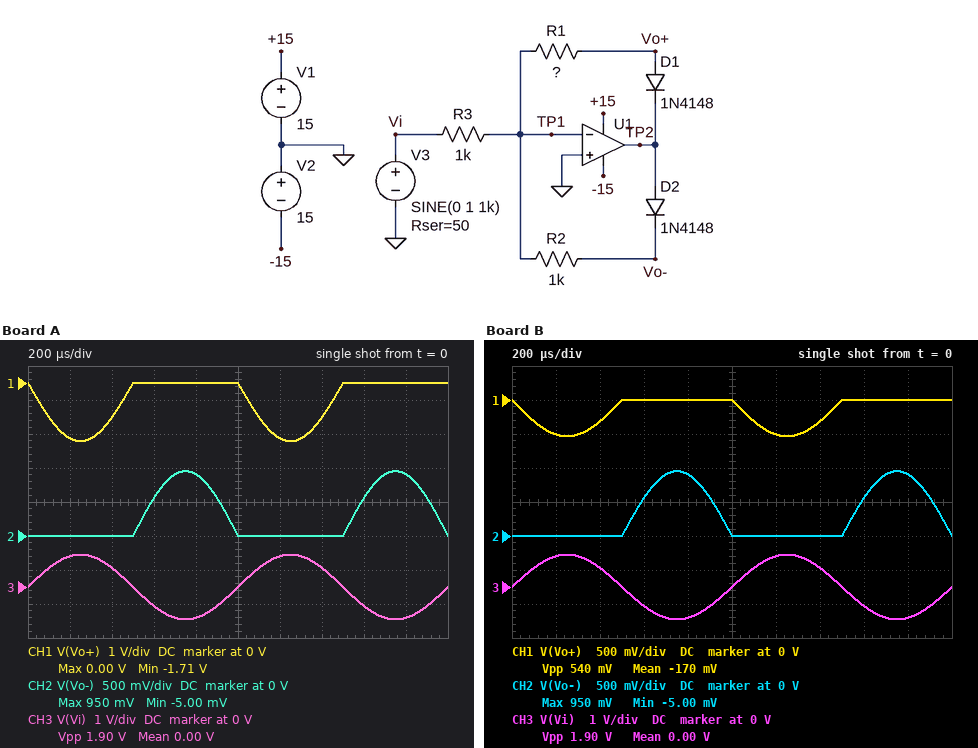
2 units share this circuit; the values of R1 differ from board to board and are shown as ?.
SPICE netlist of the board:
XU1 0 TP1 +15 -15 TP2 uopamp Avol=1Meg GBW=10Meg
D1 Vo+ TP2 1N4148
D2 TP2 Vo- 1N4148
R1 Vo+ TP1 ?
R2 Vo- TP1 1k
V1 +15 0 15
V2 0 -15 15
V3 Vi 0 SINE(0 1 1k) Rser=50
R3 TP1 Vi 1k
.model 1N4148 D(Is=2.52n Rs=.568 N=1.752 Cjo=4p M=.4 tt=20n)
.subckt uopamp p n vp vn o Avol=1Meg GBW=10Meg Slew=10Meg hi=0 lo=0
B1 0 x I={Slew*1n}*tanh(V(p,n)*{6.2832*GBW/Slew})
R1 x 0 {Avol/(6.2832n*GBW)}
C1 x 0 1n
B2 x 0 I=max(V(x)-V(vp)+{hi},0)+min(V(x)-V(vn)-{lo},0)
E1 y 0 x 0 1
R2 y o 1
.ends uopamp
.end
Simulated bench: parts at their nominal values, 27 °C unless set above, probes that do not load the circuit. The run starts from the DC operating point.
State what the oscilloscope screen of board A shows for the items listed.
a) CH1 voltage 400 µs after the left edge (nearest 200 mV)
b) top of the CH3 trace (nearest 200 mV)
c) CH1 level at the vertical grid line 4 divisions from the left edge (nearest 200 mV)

-1.0 V
1.0 V
0 V
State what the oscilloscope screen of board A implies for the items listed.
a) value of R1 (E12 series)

1.8 kΩ
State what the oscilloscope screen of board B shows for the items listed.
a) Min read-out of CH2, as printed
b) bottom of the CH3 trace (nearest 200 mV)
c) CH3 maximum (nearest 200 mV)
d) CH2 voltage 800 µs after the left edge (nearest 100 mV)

-5.00 mV
-1.0 V
1.0 V
900 mV
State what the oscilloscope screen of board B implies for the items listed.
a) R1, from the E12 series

560 Ω
